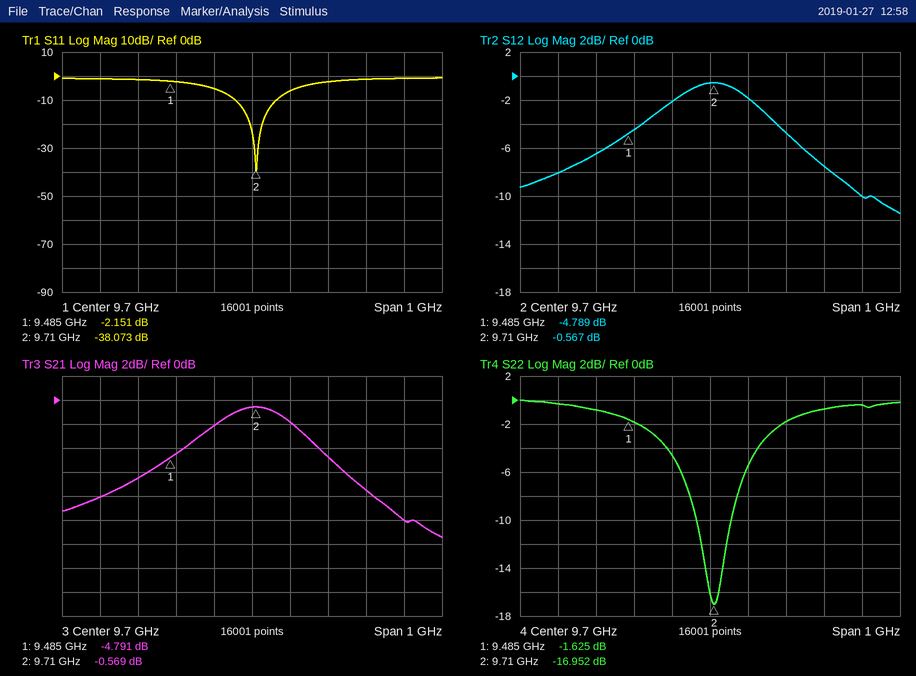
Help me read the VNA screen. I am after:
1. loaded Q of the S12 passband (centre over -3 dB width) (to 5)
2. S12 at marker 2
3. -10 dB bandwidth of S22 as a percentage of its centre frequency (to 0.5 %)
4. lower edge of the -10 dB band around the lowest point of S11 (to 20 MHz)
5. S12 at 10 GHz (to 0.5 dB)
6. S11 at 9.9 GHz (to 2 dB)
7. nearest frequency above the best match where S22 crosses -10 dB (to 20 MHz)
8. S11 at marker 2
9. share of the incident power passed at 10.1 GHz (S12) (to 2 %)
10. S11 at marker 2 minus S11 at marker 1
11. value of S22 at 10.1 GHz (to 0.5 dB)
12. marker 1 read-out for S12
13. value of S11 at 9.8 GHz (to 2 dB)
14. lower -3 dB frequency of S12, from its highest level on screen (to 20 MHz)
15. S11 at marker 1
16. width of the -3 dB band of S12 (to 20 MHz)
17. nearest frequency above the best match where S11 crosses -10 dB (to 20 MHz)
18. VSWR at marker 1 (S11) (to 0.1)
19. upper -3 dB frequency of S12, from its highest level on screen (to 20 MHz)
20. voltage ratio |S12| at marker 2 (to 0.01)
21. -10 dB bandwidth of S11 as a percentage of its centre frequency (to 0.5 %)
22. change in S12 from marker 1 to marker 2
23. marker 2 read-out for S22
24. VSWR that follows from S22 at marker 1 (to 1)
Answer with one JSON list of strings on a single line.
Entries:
["30", "-0.567 dB", "1.0 %", "9.66 GHz", "-7.5 dB", "-2 dB", "9.76 GHz", "-38.073 dB", "10 %", "-35.922 dB", "-0.5 dB", "-4.789 dB", "-6 dB", "9.54 GHz", "-2.151 dB", "320 MHz", "9.76 GHz", "8.1", "9.86 GHz", "0.94", "1.0 %", "4.222 dB", "-16.952 dB", "11"]
